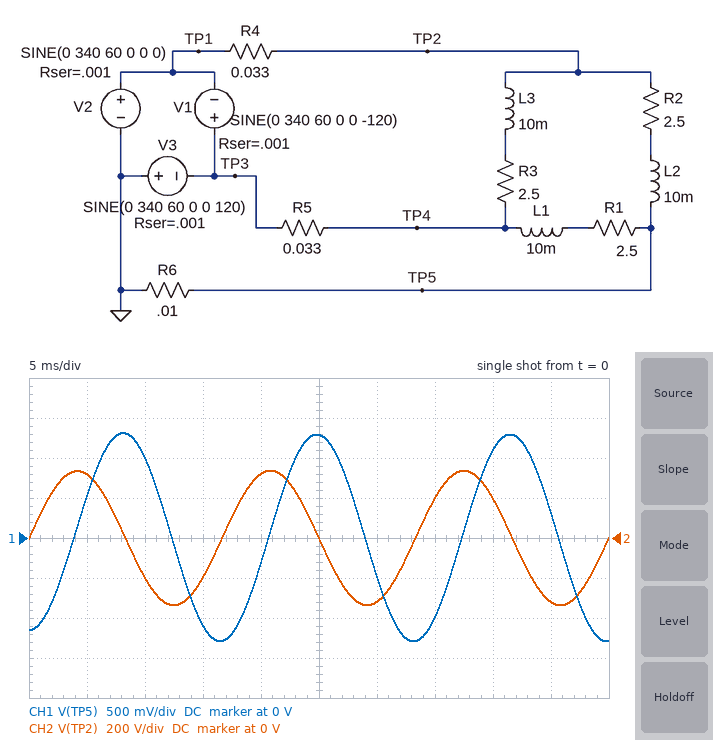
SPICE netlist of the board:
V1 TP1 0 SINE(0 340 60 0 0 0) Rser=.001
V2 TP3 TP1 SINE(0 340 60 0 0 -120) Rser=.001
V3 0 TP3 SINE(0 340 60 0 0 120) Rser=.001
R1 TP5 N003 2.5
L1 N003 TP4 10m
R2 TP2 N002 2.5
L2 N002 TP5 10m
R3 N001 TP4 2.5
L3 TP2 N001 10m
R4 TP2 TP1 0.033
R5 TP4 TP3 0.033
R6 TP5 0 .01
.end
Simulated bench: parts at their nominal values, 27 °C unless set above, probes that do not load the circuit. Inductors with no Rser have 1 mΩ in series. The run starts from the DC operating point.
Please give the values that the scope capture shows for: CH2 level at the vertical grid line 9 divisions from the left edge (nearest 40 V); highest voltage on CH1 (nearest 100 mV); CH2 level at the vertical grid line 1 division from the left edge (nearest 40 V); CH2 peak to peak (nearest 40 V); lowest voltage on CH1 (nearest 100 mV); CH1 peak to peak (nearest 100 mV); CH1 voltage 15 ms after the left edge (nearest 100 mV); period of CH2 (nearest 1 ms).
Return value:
-320 V
1.3 V
320 V
680 V
-1.3 V
2.6 V
-1.1 V
17 ms
